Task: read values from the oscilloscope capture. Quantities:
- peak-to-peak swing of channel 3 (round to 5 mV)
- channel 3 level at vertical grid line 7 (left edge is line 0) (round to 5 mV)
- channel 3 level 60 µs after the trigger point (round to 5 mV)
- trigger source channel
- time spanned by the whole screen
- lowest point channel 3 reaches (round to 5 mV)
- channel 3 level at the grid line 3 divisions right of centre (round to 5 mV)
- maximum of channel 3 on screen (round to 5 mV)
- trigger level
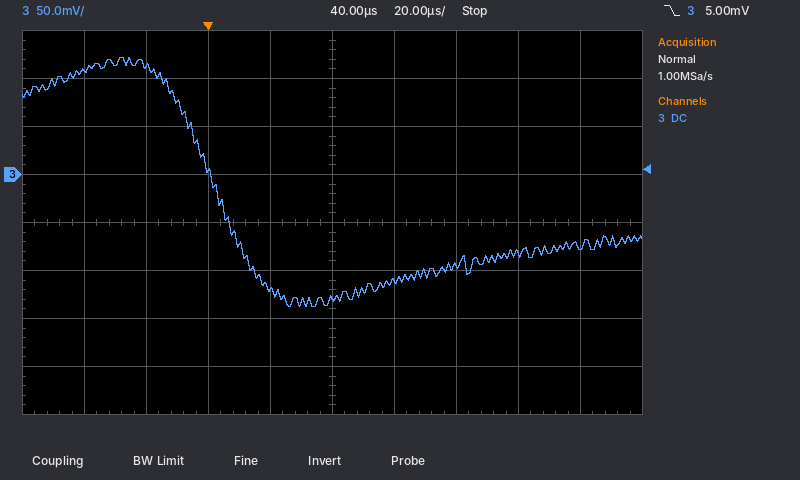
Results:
260 mV
-95 mV
-110 mV
channel 3
200 µs
-140 mV
-80 mV
120 mV
5.00 mV
